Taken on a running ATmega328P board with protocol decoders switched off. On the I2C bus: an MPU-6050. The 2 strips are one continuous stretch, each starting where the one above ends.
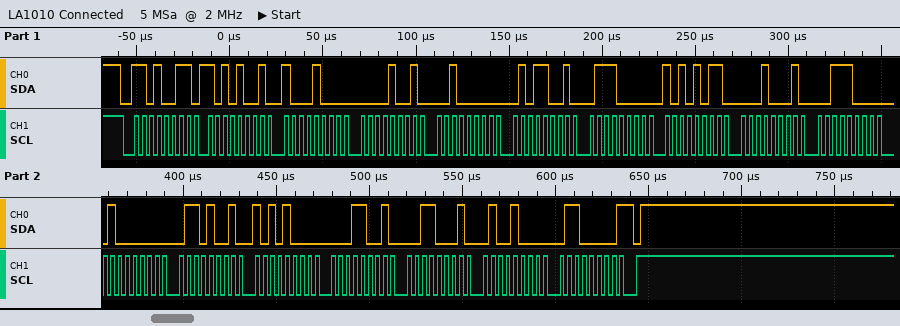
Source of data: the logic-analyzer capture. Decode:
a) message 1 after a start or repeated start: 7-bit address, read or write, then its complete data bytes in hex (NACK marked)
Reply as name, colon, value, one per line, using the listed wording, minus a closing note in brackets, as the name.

message 1 after a start or repeated start: 7-bit address, read or write, then its complete data bytes in hex: 0x69 read: A9 88 09 20 59 70 AB 11 38 40 69 A8 19 31 48 60 NACK
